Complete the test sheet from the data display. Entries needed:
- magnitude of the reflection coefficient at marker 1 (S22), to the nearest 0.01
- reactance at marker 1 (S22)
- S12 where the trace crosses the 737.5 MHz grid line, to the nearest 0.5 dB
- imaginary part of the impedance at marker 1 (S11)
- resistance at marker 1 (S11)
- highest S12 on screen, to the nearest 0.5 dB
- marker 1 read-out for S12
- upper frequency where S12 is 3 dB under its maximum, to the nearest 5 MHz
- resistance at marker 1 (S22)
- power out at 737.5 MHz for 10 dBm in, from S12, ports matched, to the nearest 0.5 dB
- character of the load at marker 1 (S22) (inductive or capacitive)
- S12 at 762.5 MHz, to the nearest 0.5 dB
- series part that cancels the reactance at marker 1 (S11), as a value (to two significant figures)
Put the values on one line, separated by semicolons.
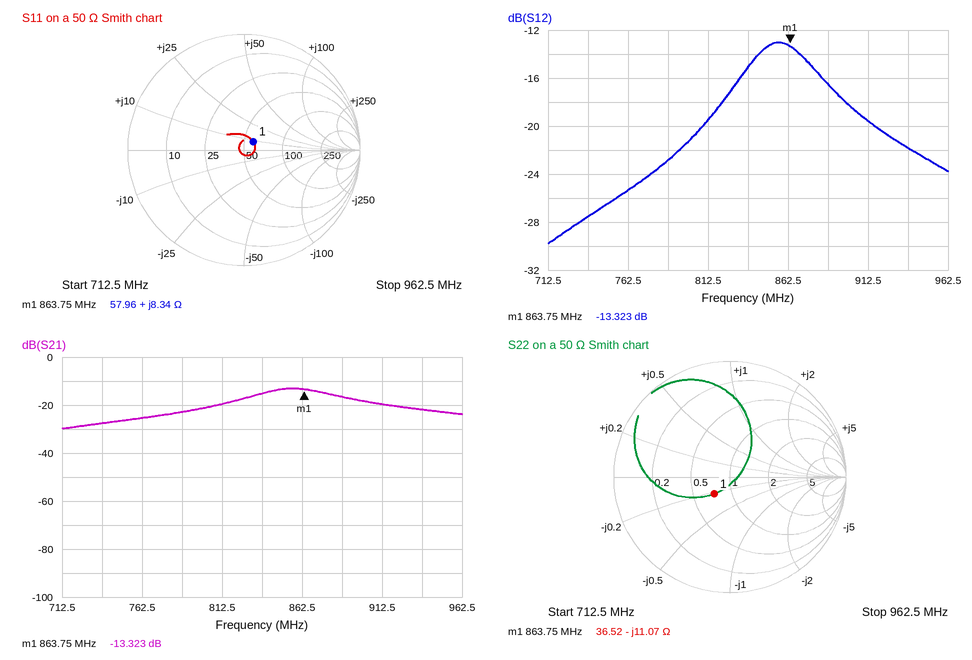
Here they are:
0.20; -11.07 Ω; -27.5 dB; +8.34 Ω; 57.96 Ω; -13.0 dB; -13.323 dB; 885 MHz; 36.52 Ω; -17.5 dBm; capacitive; -25.5 dB; 22 pF
